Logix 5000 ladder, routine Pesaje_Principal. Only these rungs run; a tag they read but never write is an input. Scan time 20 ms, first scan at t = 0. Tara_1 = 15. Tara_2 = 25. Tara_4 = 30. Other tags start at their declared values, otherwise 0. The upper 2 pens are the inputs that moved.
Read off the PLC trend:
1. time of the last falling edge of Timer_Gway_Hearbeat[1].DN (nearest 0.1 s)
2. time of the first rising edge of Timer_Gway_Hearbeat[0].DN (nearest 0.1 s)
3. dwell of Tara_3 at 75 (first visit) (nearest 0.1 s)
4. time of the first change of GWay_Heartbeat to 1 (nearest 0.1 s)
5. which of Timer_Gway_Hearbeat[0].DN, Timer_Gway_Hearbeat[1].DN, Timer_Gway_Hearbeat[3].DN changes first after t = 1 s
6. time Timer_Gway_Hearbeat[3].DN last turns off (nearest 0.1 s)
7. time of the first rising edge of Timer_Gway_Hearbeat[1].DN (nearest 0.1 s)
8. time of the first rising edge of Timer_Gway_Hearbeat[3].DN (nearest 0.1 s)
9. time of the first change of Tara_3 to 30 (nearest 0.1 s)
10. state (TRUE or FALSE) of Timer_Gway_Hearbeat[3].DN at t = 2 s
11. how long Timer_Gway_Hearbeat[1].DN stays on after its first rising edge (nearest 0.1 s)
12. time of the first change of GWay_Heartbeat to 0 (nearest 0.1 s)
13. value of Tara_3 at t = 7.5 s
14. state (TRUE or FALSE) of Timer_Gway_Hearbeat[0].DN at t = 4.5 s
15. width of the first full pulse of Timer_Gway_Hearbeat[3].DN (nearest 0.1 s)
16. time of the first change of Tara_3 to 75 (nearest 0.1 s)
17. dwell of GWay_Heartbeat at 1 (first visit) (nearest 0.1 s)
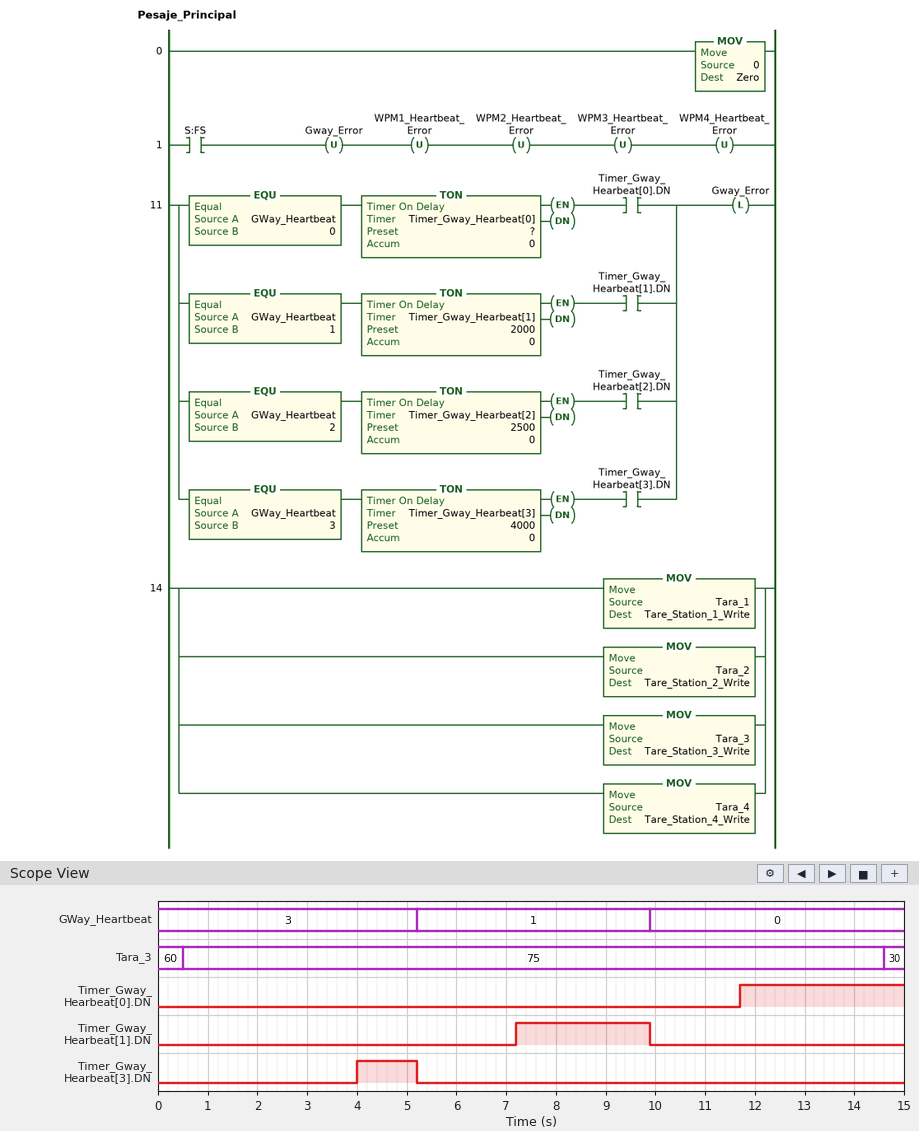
9.9 s
11.7 s
14.1 s
5.2 s
Timer_Gway_Hearbeat[3].DN
5.2 s
7.2 s
4.0 s
14.6 s
FALSE
2.7 s
9.9 s
75
FALSE
1.2 s
0.5 s
4.7 s
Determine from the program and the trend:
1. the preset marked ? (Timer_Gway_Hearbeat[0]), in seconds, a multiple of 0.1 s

1.8 s
